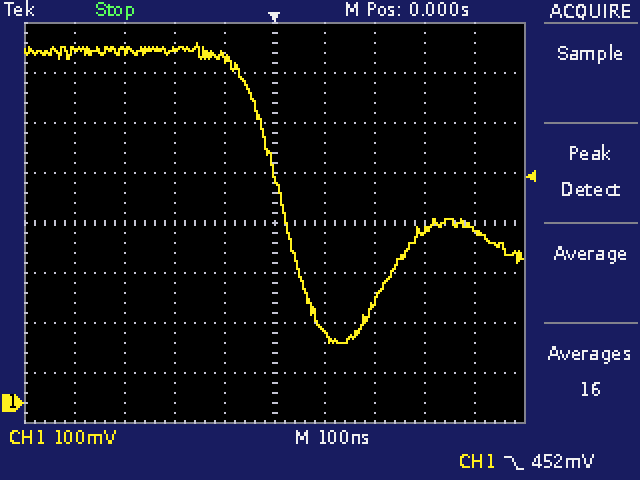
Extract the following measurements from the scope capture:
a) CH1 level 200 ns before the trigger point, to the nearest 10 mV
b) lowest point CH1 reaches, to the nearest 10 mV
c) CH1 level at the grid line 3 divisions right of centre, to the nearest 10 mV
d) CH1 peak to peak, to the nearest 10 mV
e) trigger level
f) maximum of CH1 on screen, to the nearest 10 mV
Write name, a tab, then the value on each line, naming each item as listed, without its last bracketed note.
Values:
CH1 level 200 ns before the trigger point, to the nearest 10 mV	710 mV
lowest point CH1 reaches, to the nearest 10 mV	120 mV
CH1 level at the grid line 3 divisions right of centre, to the nearest 10 mV	340 mV
CH1 peak to peak, to the nearest 10 mV	600 mV
trigger level	452 mV
maximum of CH1 on screen, to the nearest 10 mV	720 mV
